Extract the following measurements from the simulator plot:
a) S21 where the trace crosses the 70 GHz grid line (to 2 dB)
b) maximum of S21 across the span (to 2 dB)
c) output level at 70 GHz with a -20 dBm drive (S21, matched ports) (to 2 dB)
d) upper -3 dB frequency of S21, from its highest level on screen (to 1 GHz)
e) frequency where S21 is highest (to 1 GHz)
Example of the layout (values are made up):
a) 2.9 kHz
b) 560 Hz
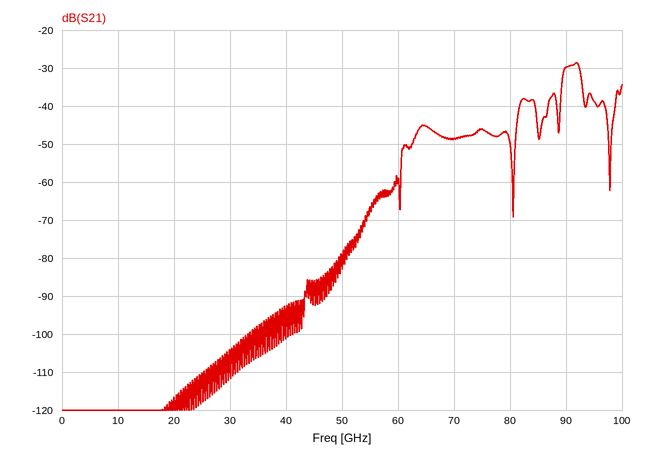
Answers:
a) -48 dB
b) -28 dB
c) -68 dBm
d) 93 GHz
e) 92 GHz
